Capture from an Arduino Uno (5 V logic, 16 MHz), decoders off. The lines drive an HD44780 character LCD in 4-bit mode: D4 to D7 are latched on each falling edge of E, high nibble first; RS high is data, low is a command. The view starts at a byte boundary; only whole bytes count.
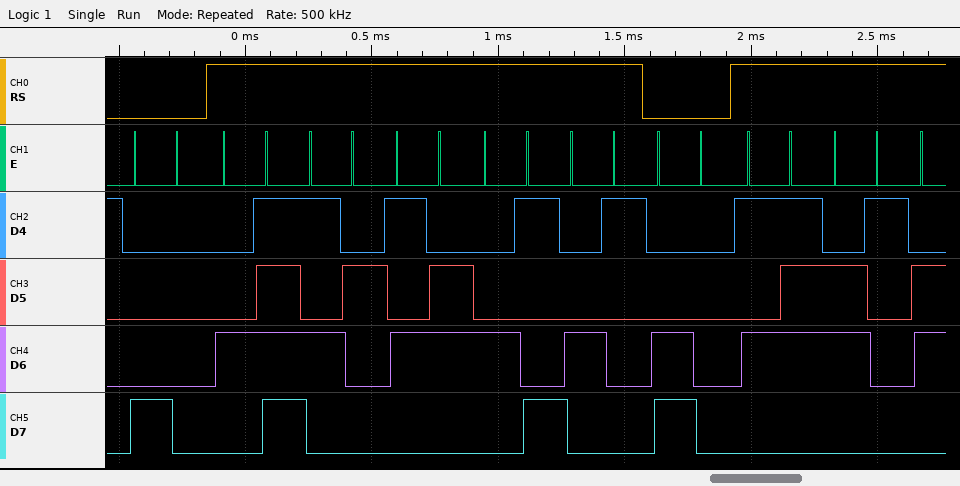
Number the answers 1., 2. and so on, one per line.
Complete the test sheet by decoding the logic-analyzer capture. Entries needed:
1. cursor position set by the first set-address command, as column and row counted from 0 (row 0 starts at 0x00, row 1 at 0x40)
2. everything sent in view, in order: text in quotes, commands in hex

1. column 0, row 0
2. 0x80 "ORVIA" 0xC0 "Wa"
